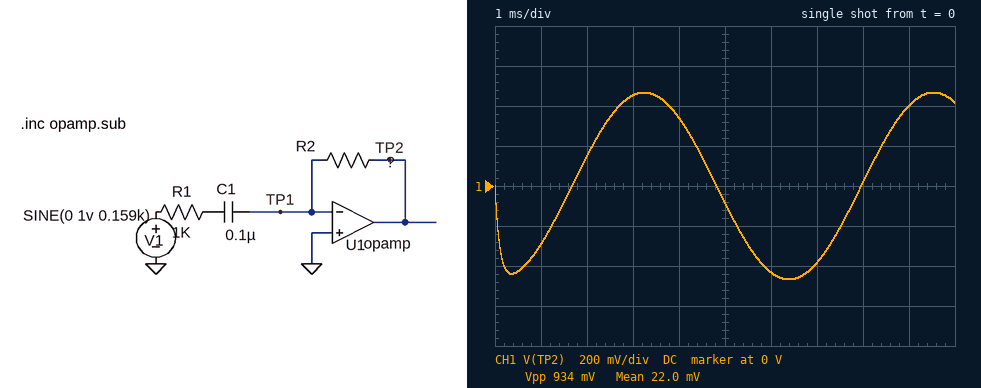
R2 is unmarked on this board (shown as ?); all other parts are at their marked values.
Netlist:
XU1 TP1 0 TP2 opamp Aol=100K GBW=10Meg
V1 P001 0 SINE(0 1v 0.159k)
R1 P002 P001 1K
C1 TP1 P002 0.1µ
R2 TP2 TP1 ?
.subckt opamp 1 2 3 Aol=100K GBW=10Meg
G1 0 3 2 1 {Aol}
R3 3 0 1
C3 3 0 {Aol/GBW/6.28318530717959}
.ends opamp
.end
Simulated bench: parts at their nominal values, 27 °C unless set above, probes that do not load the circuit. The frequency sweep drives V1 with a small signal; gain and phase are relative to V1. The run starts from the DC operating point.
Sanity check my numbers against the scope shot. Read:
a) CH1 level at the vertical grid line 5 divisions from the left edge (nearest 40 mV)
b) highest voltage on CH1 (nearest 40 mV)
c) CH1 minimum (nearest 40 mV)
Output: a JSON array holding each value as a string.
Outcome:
["-80 mV", "480 mV", "-480 mV"]
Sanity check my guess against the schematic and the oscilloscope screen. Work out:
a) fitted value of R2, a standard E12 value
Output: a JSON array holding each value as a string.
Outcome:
["4.7 kΩ"]
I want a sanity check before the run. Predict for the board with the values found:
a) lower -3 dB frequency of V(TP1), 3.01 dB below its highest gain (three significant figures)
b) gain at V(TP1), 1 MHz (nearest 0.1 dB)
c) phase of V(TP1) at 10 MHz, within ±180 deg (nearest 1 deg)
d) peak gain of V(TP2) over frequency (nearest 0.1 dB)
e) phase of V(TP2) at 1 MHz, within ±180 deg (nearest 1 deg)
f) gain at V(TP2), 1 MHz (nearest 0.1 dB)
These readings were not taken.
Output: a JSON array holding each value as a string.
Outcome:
["1.75 MHz", "-7.8 dB", "10 deg", "13.4 dB", "150 deg", "12.2 dB"]
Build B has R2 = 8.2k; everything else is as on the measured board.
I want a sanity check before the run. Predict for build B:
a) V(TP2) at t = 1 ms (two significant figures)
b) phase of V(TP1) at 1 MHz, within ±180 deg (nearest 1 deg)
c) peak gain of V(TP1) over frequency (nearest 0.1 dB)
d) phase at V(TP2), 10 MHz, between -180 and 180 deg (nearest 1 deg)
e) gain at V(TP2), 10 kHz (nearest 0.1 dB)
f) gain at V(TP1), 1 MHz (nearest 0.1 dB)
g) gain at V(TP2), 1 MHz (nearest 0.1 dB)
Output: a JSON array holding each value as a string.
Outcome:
["-510 mV", "47 deg", "-1.0 dB", "96 deg", "18.2 dB", "-4.4 dB", "15.6 dB"]
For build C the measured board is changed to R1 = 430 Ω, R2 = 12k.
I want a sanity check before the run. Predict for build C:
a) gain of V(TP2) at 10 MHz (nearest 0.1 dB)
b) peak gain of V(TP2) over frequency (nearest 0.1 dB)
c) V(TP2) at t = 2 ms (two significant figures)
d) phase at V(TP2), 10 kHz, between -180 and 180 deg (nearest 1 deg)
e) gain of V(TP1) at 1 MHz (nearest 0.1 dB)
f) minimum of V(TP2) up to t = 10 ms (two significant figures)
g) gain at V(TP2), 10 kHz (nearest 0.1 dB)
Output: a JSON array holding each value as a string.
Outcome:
["-0.3 dB", "28.9 dB", "450 mV", "-161 deg", "-0.8 dB", "-1.2 V", "28.4 dB"]
